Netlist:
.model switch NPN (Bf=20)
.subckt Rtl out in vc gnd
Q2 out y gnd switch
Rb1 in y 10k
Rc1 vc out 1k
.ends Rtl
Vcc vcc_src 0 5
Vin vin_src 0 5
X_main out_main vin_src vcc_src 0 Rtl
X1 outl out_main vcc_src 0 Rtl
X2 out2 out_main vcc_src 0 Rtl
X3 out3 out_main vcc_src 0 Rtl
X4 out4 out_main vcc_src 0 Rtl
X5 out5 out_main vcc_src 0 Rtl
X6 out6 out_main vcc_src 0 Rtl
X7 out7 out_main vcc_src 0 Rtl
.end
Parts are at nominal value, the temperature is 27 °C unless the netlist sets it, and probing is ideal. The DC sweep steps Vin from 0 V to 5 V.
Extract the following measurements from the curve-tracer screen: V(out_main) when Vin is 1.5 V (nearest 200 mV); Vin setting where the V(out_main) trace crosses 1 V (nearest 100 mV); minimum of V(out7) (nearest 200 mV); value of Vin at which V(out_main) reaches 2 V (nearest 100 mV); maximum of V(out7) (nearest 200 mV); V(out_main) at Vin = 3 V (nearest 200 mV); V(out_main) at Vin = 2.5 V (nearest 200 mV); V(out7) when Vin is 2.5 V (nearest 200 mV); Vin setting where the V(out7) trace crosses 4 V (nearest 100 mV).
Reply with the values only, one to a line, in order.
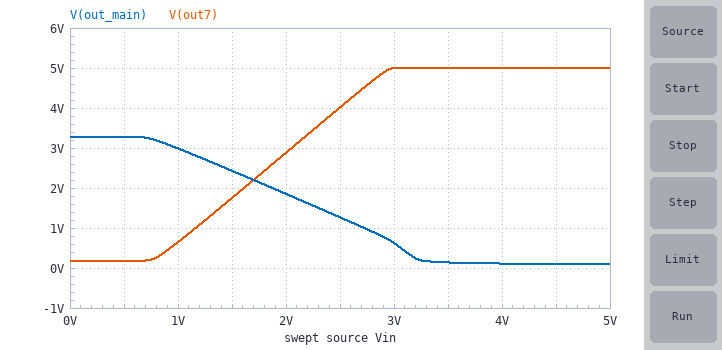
2.4 V
2.7 V
200 mV
1.9 V
5.0 V
600 mV
1.2 V
4.0 V
2.5 V
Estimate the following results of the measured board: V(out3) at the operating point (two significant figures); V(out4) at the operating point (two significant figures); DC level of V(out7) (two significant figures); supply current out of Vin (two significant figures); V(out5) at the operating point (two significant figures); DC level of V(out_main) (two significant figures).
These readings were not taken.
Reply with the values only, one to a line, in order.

5.0 V
5.0 V
5.0 V
420 µA
5.0 V
91 mV
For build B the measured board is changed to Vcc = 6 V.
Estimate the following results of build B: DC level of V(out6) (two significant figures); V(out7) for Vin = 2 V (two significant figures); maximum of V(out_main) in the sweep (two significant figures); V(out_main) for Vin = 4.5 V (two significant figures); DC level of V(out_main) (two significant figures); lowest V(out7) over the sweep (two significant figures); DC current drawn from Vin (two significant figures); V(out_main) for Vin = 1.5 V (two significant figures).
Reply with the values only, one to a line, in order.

6.0 V
2.7 V
3.9 V
120 mV
100 mV
160 mV
420 µA
3.0 V
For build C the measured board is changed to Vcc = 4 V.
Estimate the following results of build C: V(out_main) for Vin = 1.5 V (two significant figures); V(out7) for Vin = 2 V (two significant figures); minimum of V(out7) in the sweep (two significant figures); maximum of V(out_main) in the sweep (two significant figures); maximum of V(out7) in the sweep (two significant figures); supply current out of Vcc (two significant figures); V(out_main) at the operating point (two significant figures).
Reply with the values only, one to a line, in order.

1.8 V
3.0 V
250 mV
2.7 V
4.0 V
3.9 mA
79 mV
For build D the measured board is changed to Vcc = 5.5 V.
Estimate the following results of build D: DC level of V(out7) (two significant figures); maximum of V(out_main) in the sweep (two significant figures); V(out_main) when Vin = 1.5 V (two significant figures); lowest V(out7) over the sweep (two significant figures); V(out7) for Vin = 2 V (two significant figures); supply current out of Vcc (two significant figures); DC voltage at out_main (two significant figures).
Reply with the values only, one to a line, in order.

5.5 V
3.6 V
2.7 V
170 mV
2.8 V
5.4 mA
97 mV
